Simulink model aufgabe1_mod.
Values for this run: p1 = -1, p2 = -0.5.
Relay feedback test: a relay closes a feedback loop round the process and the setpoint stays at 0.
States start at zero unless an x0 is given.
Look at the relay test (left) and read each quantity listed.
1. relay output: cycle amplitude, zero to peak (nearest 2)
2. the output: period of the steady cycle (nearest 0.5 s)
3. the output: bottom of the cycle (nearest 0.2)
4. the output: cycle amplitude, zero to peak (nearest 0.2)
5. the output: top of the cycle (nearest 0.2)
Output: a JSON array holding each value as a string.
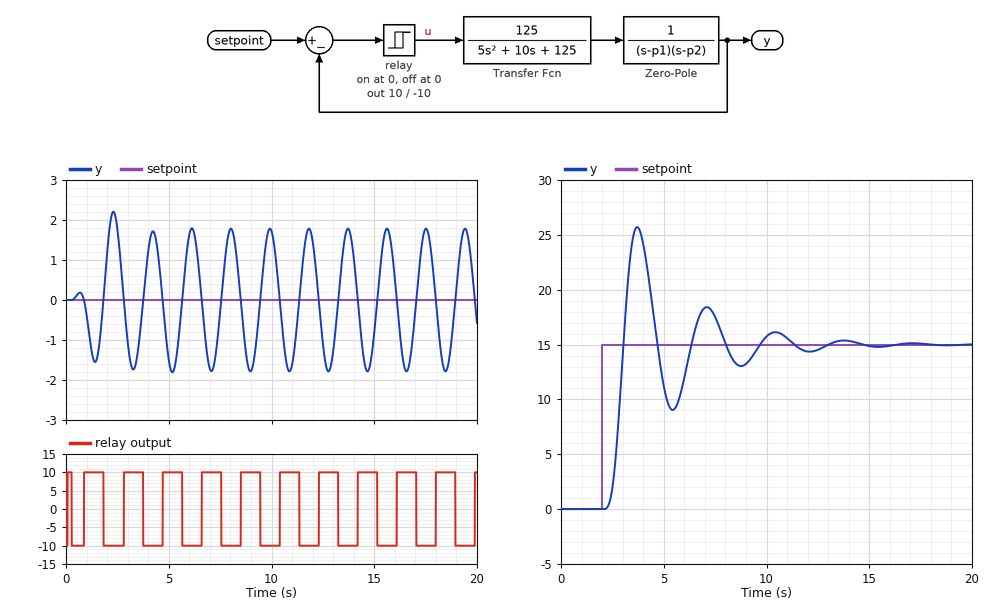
["10", "2.0 s", "-1.8", "1.8", "1.8"]
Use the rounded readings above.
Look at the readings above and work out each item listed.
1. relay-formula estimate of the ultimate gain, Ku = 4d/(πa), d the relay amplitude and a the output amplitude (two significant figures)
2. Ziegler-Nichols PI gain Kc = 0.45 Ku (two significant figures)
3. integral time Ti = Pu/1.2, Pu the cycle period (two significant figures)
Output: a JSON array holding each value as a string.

["7.1", "3.2", "1.7 s"]
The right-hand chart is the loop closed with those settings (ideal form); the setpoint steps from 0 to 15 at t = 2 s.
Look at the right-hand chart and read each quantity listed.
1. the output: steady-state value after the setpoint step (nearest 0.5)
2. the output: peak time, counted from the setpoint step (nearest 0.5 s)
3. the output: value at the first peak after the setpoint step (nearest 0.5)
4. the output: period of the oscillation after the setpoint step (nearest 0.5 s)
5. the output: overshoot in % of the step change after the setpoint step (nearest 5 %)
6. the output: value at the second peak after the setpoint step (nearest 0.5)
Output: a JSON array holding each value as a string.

["15.0", "1.5 s", "25.5", "3.5 s", "70 %", "18.5"]
